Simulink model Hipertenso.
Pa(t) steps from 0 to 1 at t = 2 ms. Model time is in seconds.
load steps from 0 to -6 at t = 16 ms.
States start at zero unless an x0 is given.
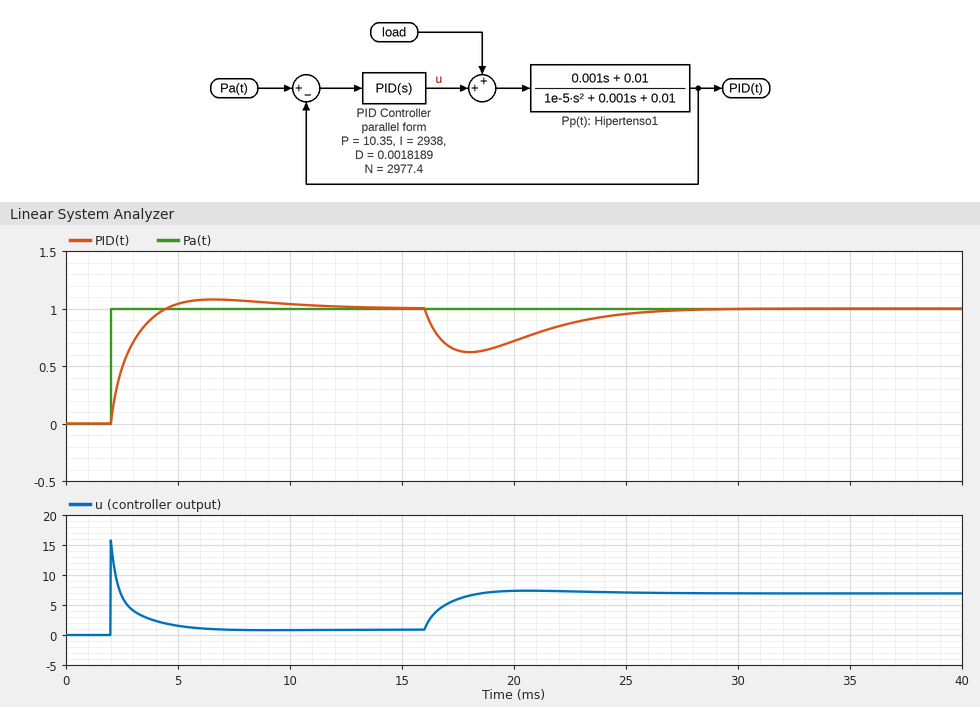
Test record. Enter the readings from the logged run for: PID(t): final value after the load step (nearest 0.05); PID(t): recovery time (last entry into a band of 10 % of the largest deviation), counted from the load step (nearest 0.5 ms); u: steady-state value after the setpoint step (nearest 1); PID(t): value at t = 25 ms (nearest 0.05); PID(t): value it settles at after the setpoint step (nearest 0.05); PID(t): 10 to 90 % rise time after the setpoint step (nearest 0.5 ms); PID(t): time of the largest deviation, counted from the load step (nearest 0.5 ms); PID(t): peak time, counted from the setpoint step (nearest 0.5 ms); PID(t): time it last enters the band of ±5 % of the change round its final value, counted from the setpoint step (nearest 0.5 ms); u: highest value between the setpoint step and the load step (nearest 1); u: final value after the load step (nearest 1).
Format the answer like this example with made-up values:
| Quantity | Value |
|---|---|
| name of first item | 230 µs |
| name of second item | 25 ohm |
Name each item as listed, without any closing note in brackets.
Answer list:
| Quantity | Value |
|---|---|
| PID(t): final value after the load step | 1.00 |
| PID(t): recovery time (last entry into a band of 10 % of the largest deviation), counted from the load step | 9.5 ms |
| u: steady-state value after the setpoint step | 1 |
| PID(t): value at t = 25 ms | 0.95 |
| PID(t): value it settles at after the setpoint step | 1.00 |
| PID(t): 10 to 90 % rise time after the setpoint step | 1.5 ms |
| PID(t): time of the largest deviation, counted from the load step | 2.0 ms |
| PID(t): peak time, counted from the setpoint step | 4.5 ms |
| PID(t): time it last enters the band of ±5 % of the change round its final value, counted from the setpoint step | 7.0 ms |
| u: highest value between the setpoint step and the load step | 16 |
| u: final value after the load step | 7 |
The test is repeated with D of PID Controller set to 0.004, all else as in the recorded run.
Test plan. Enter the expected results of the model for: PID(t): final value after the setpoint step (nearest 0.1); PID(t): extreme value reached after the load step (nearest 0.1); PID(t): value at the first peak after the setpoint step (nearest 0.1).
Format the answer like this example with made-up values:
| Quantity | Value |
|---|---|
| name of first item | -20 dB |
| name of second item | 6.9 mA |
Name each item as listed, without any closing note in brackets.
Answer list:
| Quantity | Value |
|---|---|
| PID(t): final value after the setpoint step | 1.0 |
| PID(t): extreme value reached after the load step | 0.6 |
| PID(t): value at the first peak after the setpoint step | 1.1 |
